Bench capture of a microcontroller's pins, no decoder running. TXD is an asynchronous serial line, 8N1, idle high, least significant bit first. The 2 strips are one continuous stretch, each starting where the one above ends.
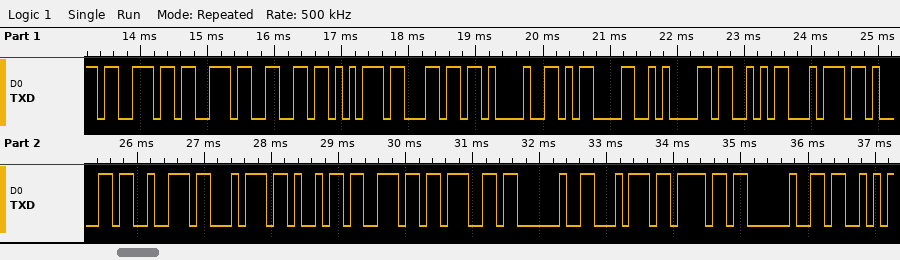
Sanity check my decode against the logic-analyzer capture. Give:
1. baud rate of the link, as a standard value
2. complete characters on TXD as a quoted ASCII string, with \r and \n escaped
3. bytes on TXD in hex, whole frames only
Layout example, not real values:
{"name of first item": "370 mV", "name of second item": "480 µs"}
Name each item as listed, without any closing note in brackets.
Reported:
{"baud rate of the link, as a standard value": "9600 baud", "complete characters on TXD as a quoted ASCII string, with \\r and \\n escaped": "\"ssful!\\r\\nStarting to S\"", "bytes on TXD in hex, whole frames only": "73 73 66 75 6C 21 0D 0A 53 74 61 72 74 69 6E 67 20 74 6F 20 53"}
